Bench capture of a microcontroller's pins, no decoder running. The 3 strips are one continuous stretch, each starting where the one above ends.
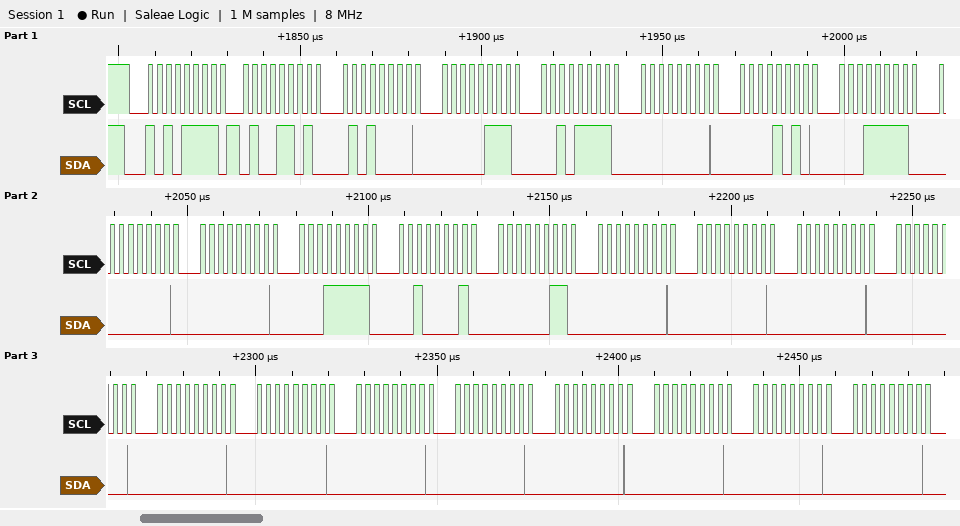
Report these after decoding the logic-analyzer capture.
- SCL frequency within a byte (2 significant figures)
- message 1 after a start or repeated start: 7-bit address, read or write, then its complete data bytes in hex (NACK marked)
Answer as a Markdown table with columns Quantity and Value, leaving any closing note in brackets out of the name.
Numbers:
| Quantity | Value |
|---|---|
| SCL frequency within a byte | 400 kHz |
| message 1 after a start or repeated start: 7-bit address, read or write, then its complete data bytes in hex | 0x57 read: 4D 50 07 2F 00 0A 1F 00 00 1F 21 03 00 00 00 00 00 00 00 00 00 00 00 00 |
